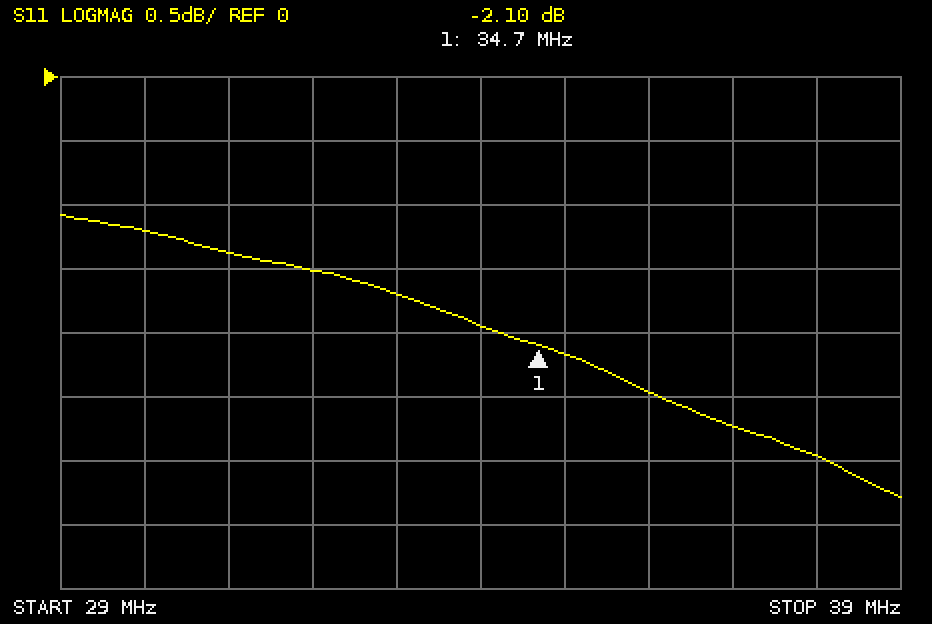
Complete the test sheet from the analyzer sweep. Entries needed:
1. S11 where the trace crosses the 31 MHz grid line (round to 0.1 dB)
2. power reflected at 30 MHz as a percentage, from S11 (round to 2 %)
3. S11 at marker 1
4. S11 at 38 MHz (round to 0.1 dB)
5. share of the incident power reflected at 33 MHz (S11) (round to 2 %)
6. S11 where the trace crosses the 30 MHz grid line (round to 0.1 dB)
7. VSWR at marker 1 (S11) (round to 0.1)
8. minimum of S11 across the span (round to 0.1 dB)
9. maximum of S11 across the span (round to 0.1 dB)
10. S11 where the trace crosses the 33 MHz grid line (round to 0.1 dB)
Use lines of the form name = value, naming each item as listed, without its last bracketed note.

S11 where the trace crosses the 31 MHz grid line = -1.4 dB
power reflected at 30 MHz as a percentage, from S11 = 76 %
S11 at marker 1 = -2.10 dB
S11 at 38 MHz = -3.0 dB
share of the incident power reflected at 33 MHz (S11) = 68 %
S11 where the trace crosses the 30 MHz grid line = -1.2 dB
VSWR at marker 1 (S11) = 8.3
minimum of S11 across the span = -3.3 dB
maximum of S11 across the span = -1.1 dB
S11 where the trace crosses the 33 MHz grid line = -1.7 dB
